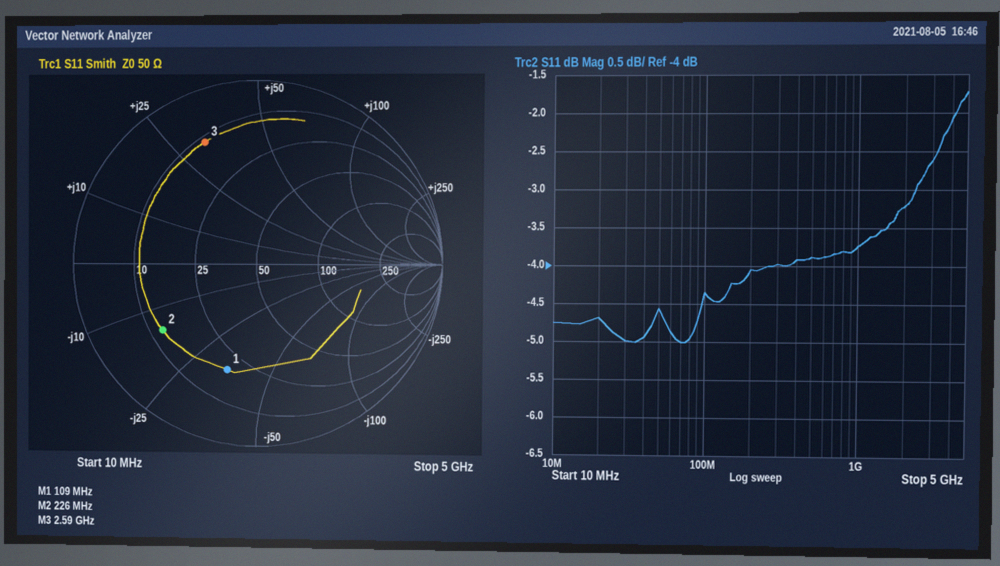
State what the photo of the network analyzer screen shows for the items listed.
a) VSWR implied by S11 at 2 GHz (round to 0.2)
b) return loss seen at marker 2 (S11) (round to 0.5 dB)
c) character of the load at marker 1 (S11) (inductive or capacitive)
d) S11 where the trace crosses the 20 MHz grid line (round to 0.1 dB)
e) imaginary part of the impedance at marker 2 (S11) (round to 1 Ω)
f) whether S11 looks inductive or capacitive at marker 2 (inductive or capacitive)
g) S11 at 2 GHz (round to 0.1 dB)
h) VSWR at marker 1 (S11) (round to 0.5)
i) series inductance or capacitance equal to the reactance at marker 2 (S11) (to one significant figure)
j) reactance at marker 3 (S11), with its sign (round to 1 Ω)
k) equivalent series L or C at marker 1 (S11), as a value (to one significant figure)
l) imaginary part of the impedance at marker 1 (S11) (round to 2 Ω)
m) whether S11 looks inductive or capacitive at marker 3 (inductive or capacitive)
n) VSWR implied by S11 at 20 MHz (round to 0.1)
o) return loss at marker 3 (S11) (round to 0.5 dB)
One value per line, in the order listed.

5.4
4.0 dB
capacitive
-4.7 dB
-15 Ω
capacitive
-3.2 dB
4.0
50 pF
+32 Ω
40 pF
-34 Ω
inductive
3.8
3.0 dB
